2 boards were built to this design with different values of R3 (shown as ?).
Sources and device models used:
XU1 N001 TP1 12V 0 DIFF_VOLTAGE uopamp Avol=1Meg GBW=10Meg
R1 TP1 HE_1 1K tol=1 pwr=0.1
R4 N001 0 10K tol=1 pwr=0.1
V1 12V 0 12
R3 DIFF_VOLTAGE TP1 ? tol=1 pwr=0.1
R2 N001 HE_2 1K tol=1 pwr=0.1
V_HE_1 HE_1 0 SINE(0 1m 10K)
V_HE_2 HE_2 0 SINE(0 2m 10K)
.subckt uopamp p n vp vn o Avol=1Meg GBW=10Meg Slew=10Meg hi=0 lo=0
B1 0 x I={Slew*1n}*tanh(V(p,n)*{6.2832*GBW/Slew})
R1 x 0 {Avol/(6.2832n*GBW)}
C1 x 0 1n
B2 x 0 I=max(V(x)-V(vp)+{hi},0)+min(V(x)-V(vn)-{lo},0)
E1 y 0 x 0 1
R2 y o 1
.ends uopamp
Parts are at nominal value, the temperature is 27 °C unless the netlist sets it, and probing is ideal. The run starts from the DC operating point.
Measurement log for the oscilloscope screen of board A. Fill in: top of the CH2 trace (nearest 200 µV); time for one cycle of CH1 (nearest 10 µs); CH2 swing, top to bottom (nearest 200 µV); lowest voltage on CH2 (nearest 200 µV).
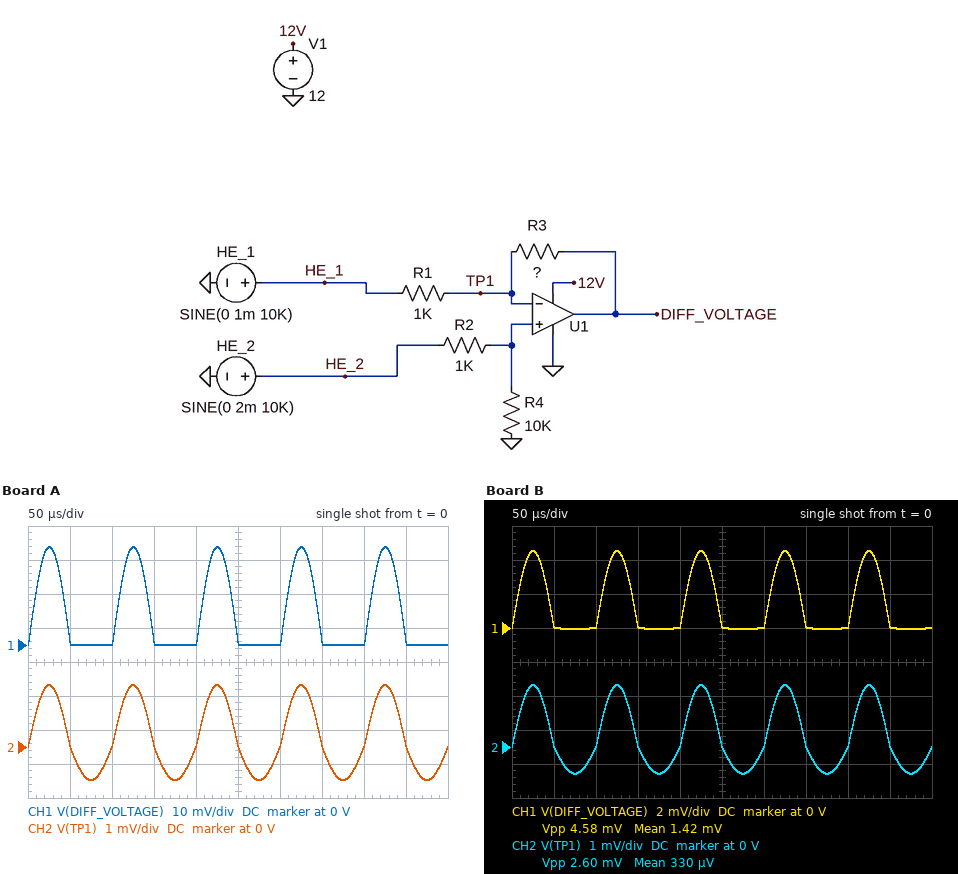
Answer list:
1.8 mV
100 µs
2.8 mV
-1.0 mV
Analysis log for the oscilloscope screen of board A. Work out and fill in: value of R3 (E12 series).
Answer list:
33 kΩ
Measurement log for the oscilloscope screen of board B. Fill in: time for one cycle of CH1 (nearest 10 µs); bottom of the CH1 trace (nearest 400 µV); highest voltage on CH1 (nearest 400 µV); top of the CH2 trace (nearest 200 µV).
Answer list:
100 µs
0 V
4.4 mV
1.8 mV
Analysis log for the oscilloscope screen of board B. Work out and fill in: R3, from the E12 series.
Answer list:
3.3 kΩ
